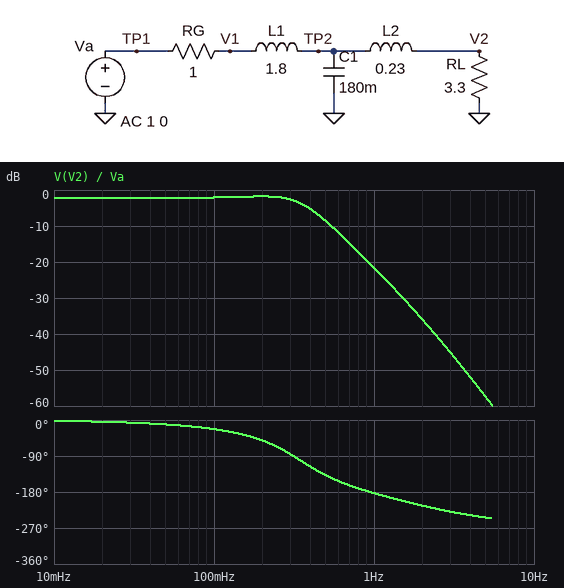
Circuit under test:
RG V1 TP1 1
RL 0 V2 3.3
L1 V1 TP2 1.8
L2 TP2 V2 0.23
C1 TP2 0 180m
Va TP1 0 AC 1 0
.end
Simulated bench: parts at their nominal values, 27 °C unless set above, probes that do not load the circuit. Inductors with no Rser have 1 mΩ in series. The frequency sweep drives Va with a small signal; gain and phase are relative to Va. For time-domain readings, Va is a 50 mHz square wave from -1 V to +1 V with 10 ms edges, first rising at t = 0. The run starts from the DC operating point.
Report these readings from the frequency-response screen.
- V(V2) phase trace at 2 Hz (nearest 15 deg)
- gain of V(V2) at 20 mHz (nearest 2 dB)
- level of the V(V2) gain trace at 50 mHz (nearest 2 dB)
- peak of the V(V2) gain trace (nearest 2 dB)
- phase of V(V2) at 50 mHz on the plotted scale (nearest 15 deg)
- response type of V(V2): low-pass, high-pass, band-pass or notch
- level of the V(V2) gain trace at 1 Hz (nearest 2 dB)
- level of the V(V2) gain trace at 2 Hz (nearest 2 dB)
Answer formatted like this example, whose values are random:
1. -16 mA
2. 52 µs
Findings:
1. -210 deg
2. -2 dB
3. -2 dB
4. -2 dB
5. -15 deg
6. low-pass
7. -22 dB
8. -36 dB
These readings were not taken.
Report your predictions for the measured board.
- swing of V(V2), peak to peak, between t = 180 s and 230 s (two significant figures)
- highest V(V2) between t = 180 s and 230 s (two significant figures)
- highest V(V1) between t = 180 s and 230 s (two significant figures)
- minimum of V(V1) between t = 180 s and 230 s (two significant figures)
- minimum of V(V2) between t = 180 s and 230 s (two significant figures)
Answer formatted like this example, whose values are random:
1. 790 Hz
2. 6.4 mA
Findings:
1. 1.9 V
2. 940 mV
3. 1.2 V
4. -1.2 V
5. -940 mV
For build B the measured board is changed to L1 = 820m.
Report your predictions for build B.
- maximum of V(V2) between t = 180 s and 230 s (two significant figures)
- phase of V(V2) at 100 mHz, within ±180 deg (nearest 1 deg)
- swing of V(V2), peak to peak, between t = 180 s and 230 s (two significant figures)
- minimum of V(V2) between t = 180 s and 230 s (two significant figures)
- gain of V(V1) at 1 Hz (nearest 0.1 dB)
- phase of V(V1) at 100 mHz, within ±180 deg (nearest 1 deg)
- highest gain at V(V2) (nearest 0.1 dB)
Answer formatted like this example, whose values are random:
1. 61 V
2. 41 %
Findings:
1. 1.0 V
2. -14 deg
3. 2.1 V
4. -1.0 V
5. -0.3 dB
6. -2 deg
7. -1.0 dB
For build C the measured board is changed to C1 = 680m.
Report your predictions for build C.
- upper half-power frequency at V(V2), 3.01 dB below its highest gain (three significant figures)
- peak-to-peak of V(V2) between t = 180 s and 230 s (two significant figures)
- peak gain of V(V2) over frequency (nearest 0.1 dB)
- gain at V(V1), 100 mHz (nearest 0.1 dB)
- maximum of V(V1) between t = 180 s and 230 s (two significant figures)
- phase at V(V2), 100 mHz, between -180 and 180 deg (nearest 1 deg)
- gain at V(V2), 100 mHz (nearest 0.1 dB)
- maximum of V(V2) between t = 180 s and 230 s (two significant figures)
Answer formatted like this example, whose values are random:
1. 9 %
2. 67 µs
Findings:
1. 196 mHz
2. 2.1 V
3. -0.9 dB
4. -5.0 dB
5. 1.2 V
6. -45 deg
7. -1.0 dB
8. 1.0 V
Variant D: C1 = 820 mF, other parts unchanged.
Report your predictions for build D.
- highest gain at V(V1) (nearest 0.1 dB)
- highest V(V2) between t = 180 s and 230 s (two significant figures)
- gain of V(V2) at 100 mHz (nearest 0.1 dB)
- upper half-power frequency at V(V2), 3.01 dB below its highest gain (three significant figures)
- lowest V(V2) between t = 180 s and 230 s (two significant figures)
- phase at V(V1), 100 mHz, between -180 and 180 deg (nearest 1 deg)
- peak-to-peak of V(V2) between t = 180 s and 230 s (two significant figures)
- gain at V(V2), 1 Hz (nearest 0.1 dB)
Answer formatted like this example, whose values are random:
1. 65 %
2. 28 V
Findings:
1. 0 dB
2. 1.0 V
3. -1.0 dB
4. 177 mHz
5. -1.0 V
6. -11 deg
7. 2.1 V
8. -35.8 dB
